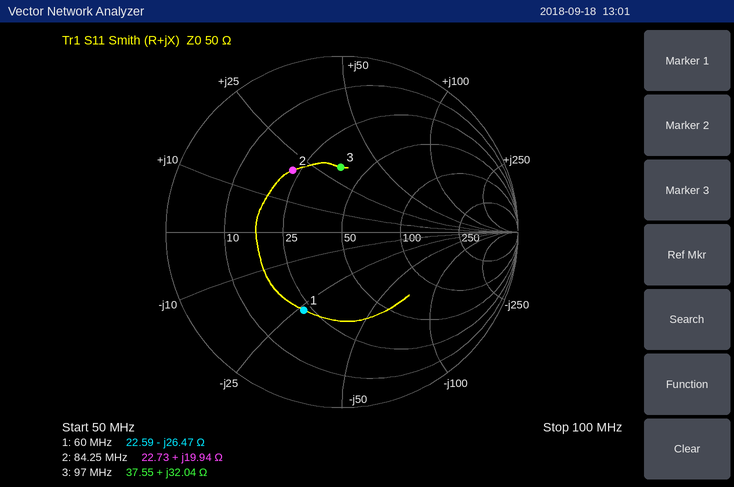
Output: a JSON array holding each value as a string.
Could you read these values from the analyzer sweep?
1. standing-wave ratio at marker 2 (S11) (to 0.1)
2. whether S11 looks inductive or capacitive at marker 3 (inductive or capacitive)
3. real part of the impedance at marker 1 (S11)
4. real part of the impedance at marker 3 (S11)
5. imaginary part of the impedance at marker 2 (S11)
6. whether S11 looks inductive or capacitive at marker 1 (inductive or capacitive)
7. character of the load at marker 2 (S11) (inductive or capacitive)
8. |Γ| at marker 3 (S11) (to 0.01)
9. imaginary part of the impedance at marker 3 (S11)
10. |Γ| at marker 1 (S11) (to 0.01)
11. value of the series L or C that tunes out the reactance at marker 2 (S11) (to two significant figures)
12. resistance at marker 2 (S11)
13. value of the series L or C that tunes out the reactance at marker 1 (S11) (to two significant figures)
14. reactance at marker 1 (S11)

["2.6", "inductive", "22.59 Ω", "37.55 Ω", "+19.94 Ω", "capacitive", "inductive", "0.37", "+32.04 Ω", "0.49", "95 pF", "22.73 Ω", "70 nH", "-26.47 Ω"]
